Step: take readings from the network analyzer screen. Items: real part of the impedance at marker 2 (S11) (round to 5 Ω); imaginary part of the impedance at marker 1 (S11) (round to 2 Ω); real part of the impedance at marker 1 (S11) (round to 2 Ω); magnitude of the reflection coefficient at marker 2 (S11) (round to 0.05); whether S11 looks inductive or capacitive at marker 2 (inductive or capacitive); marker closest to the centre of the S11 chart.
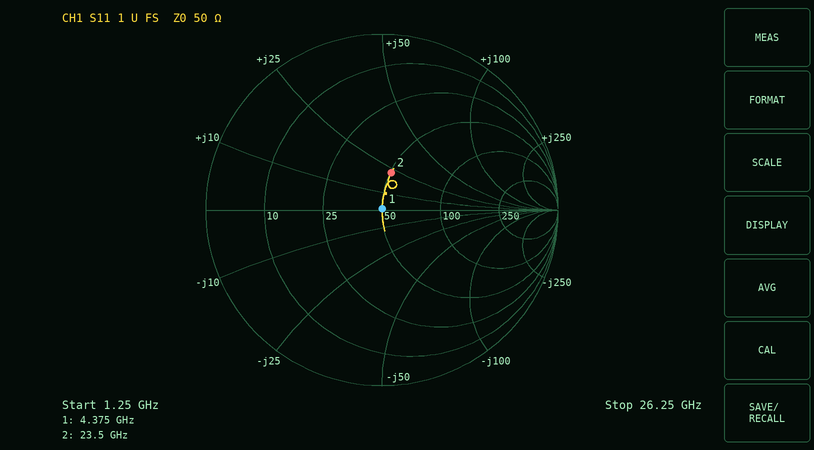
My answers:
50 Ω
0 Ω
50 Ω
0.20
inductive
marker 1
